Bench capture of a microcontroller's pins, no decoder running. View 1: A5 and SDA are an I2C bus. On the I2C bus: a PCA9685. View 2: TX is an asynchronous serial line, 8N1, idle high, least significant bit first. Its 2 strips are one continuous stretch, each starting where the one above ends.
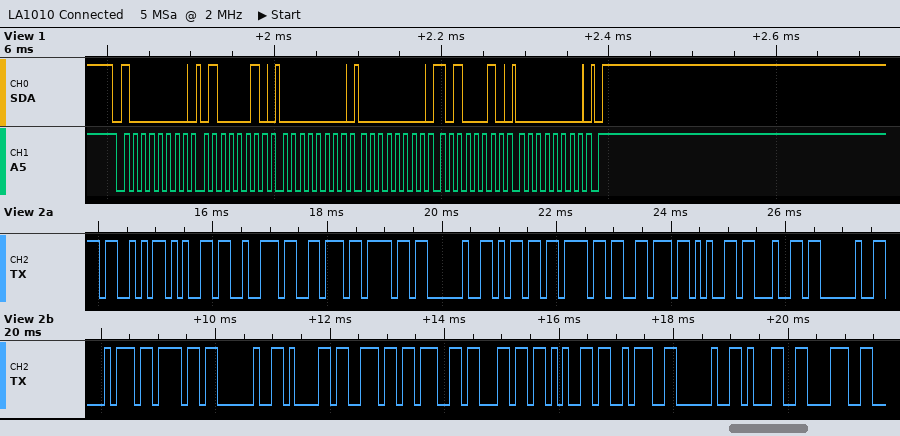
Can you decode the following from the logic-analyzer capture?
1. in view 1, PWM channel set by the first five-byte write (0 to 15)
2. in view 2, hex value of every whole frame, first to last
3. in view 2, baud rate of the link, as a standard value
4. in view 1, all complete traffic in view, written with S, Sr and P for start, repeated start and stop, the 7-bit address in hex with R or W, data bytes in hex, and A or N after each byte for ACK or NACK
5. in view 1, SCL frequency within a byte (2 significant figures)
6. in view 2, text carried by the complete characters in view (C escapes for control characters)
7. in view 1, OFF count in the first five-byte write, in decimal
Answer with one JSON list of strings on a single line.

["15", "53 65 72 76 6F 20 6D 6F 76 65 64 20 74 6F 20 61 6E 67 6C 65 3A 20 31 38", "9600 baud", "S 40W A 42 A 00 A 00 A A2 A 00 A P", "100 kHz", "\"Servo moved to angle: 18\"", "162"]
